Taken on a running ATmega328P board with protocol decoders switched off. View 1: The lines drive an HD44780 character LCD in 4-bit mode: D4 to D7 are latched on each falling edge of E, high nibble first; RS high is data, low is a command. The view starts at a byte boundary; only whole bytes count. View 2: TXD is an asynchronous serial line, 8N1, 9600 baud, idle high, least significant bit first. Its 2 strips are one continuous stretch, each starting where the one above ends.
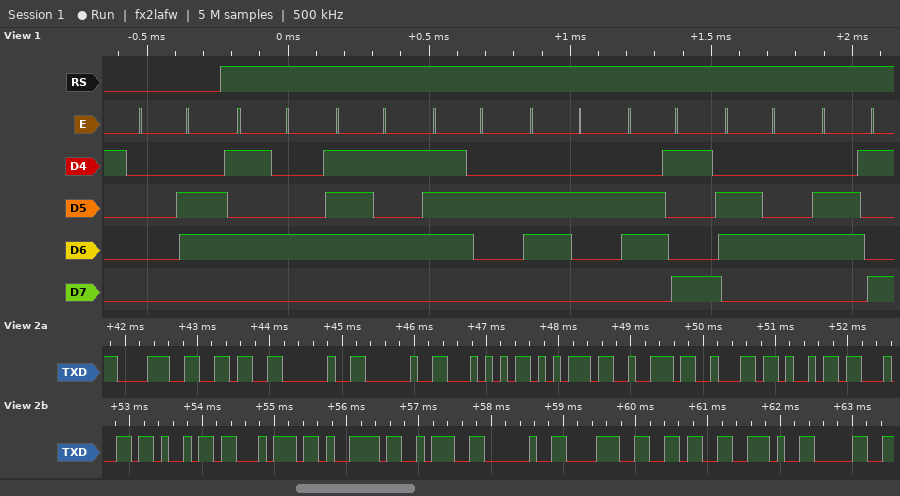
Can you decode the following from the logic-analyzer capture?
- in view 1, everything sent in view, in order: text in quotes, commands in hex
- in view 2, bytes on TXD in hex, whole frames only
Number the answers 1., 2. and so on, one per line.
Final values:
1. 0x06 "Turbidi"
2. 38 36 20 20 54 75 72 62 69 64 69 74 79 3A 20 38 36 2E 30
